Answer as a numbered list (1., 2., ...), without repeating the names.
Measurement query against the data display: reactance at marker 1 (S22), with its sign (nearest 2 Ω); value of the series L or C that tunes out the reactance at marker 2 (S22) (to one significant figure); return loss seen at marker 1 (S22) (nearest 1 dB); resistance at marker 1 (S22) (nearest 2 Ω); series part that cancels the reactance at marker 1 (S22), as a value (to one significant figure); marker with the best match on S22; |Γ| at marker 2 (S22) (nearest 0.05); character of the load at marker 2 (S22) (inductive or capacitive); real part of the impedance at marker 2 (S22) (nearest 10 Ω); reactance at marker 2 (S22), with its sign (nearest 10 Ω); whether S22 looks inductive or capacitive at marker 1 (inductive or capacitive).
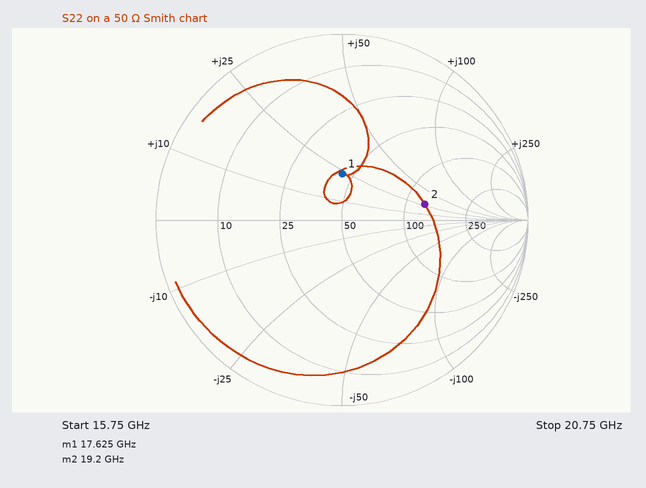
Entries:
1. +24 Ω
2. 300 fF
3. 12 dB
4. 44 Ω
5. 400 fF
6. marker 1
7. 0.45
8. inductive
9. 130 Ω
10. +30 Ω
11. inductive
